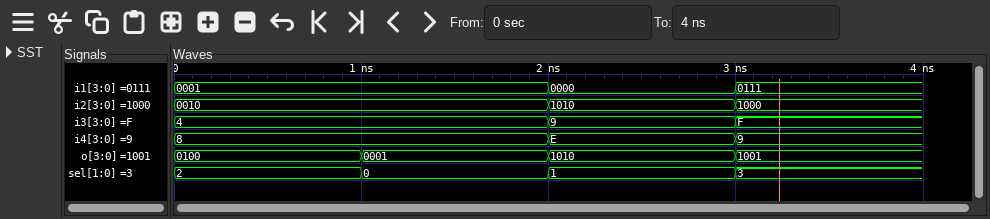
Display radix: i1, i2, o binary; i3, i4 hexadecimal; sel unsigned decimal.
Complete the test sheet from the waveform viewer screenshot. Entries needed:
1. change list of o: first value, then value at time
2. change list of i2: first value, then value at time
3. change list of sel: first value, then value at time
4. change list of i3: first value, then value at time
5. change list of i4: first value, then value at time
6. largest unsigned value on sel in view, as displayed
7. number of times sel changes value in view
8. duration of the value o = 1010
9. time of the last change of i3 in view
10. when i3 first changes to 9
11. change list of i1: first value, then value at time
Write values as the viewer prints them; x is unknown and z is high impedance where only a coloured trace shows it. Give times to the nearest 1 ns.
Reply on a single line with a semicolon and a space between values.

0100, 0001 at 1 ns, 1010 at 2 ns, 1001 at 3 ns; 0010, 1010 at 2 ns, 1000 at 3 ns; 2, 0 at 1 ns, 1 at 2 ns, 3 at 3 ns; 4, 9 at 2 ns, F at 3 ns; 8, E at 2 ns, 9 at 3 ns; 3; 3; 1 ns; 3 ns; 2 ns; 0001, 0000 at 2 ns, 0111 at 3 ns
